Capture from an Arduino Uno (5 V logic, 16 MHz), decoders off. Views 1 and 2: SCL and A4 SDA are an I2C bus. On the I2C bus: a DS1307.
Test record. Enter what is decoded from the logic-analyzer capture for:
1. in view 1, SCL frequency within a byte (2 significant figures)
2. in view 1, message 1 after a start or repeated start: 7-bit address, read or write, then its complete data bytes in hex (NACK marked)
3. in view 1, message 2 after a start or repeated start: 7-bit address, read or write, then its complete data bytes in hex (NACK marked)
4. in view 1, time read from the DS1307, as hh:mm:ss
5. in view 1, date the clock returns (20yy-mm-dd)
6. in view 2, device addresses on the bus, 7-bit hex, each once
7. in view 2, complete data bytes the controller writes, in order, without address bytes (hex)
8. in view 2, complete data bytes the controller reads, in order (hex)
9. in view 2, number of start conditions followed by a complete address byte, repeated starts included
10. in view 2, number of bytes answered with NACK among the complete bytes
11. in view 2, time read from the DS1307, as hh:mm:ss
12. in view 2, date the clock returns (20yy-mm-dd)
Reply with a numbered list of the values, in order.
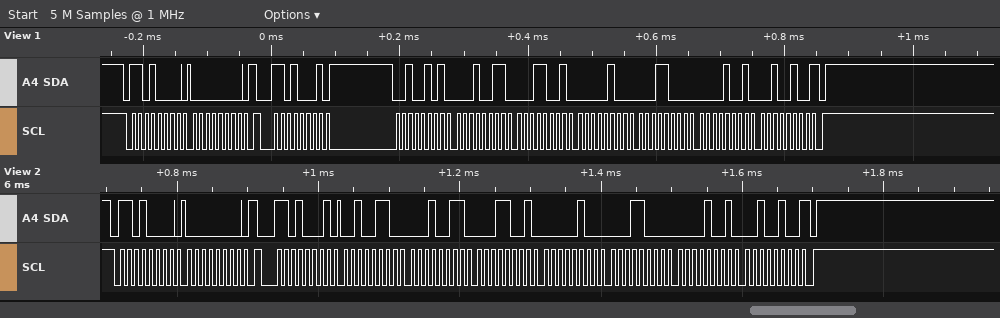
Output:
1. 100 kHz
2. 0x68 write: 00
3. 0x68 read: 25 13 19 04 18 09 24 NACK
4. 19:13:25
5. 2024-09-18
6. 0x68
7. 00
8. 26 13 19 04 18 09 24
9. 2
10. 1
11. 19:13:26
12. 2024-09-18
